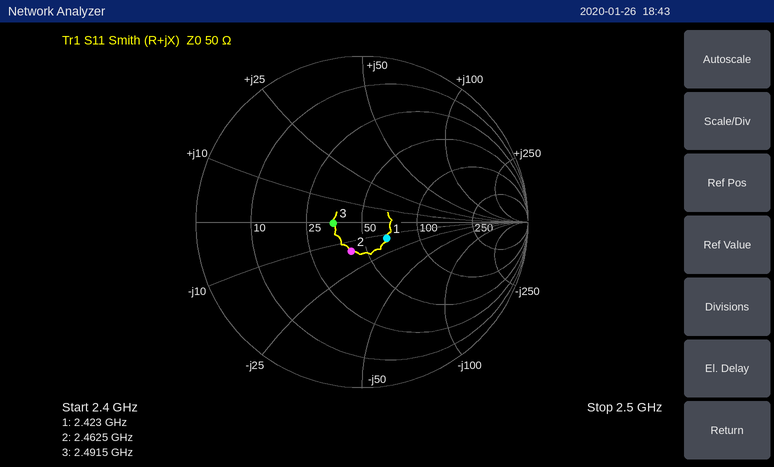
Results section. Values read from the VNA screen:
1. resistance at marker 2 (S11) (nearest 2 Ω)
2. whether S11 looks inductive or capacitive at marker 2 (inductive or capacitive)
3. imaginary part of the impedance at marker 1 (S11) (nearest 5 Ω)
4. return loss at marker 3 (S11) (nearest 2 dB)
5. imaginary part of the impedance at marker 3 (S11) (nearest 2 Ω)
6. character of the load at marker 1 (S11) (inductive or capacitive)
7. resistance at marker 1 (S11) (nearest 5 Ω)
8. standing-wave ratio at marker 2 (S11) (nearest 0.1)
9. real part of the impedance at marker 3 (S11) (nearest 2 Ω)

42 Ω
capacitive
-15 Ω
16 dB
0 Ω
capacitive
65 Ω
1.5
36 Ω
